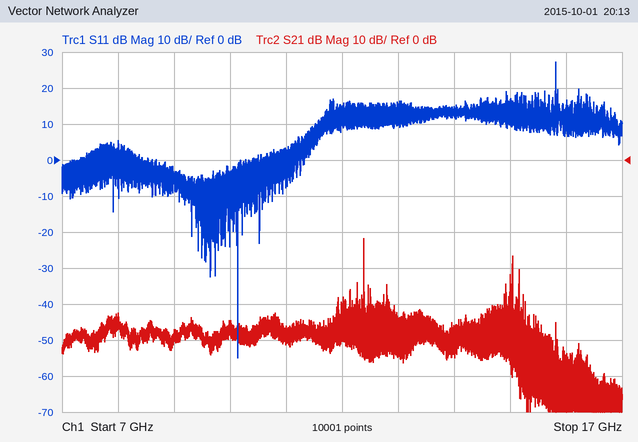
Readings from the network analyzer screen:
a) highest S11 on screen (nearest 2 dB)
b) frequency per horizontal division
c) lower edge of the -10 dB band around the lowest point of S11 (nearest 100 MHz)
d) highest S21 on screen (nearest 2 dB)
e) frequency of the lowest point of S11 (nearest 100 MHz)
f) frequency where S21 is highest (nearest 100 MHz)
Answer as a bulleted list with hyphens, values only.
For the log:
- 28 dB
- 1 GHz
- 10.1 GHz
- -22 dB
- 10.1 GHz
- 12.4 GHz
